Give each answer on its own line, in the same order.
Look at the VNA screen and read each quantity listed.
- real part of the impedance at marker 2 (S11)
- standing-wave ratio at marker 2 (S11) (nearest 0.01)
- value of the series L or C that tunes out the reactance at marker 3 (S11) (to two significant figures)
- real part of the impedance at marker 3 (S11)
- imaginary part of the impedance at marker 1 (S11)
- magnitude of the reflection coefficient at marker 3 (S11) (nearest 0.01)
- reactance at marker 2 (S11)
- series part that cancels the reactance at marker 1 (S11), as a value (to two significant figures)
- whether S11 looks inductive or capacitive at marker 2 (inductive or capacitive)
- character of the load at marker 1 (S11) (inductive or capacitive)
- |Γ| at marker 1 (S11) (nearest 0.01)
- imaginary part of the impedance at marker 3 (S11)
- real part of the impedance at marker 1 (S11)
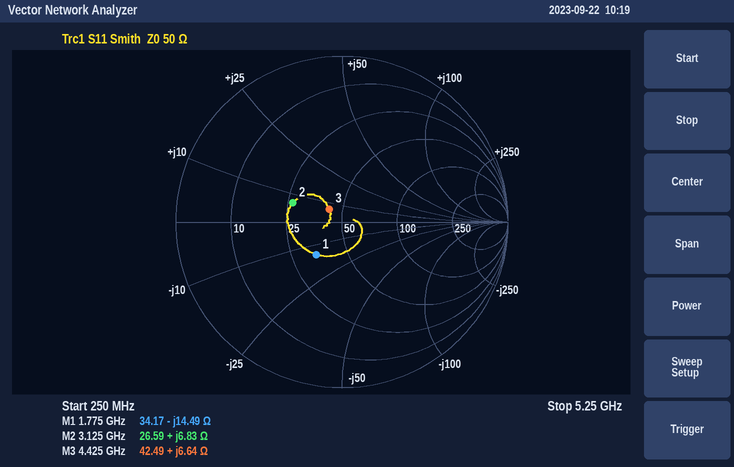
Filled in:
26.59 Ω
1.93
5.4 pF
42.49 Ω
-14.49 Ω
0.11
+6.83 Ω
1.3 nH
inductive
capacitive
0.25
+6.64 Ω
34.17 Ω
